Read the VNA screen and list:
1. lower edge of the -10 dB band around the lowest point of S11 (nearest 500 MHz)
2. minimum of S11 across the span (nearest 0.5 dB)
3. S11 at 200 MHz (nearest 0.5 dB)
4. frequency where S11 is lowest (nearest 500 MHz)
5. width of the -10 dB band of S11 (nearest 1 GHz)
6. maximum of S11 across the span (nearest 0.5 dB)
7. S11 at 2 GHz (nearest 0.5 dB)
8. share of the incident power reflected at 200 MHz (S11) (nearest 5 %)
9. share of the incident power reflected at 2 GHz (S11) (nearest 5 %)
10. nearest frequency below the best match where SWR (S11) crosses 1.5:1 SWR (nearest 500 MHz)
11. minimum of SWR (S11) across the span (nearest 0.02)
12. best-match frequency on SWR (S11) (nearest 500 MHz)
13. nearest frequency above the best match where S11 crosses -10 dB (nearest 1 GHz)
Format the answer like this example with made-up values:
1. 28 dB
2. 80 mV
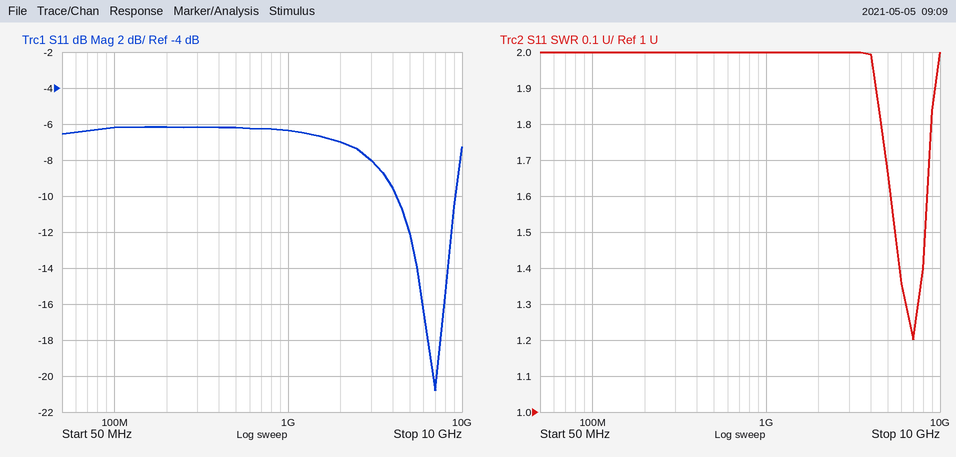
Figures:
1. 4.0 GHz
2. -21.0 dB
3. -6.0 dB
4. 7.0 GHz
5. 5 GHz
6. -6.0 dB
7. -7.0 dB
8. 25 %
9. 20 %
10. 5.5 GHz
11. 1.20
12. 7.0 GHz
13. 9 GHz
